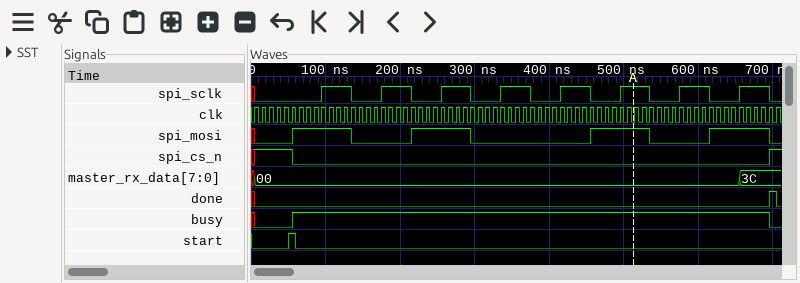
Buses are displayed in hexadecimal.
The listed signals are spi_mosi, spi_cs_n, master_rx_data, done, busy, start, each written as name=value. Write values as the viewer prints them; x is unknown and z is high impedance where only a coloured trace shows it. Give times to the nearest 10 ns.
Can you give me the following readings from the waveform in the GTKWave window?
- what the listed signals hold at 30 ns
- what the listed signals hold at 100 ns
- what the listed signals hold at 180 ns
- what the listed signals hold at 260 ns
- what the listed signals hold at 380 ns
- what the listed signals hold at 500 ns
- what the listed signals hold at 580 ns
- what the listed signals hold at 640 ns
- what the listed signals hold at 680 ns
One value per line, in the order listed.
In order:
spi_mosi=0, spi_cs_n=1, master_rx_data=00, done=0, busy=0, start=0
spi_mosi=1, spi_cs_n=0, master_rx_data=00, done=0, busy=1, start=0
spi_mosi=0, spi_cs_n=0, master_rx_data=00, done=0, busy=1, start=0
spi_mosi=1, spi_cs_n=0, master_rx_data=00, done=0, busy=1, start=0
spi_mosi=0, spi_cs_n=0, master_rx_data=00, done=0, busy=1, start=0
spi_mosi=1, spi_cs_n=0, master_rx_data=00, done=0, busy=1, start=0
spi_mosi=0, spi_cs_n=0, master_rx_data=00, done=0, busy=1, start=0
spi_mosi=1, spi_cs_n=0, master_rx_data=00, done=0, busy=1, start=0
spi_mosi=1, spi_cs_n=0, master_rx_data=3C, done=0, busy=1, start=0
